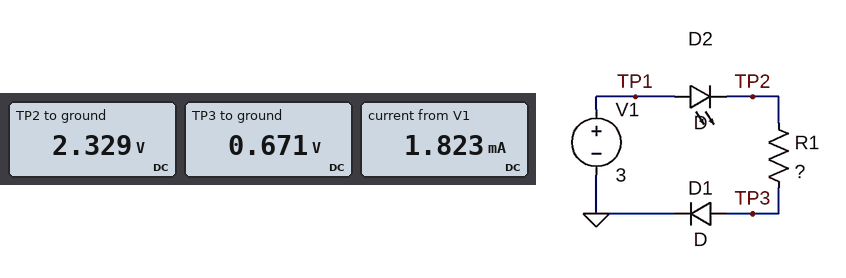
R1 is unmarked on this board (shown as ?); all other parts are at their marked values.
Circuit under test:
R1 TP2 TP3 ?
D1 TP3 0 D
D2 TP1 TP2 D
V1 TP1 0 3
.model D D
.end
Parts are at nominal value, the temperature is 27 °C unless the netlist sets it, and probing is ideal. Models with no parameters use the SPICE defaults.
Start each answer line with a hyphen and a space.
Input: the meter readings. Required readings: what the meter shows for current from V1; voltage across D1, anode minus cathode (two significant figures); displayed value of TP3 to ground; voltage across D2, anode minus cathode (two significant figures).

- 1.823 mA
- 670 mV
- 0.671 V
- 670 mV
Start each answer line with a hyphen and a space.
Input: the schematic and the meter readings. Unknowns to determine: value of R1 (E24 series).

- 910 Ω
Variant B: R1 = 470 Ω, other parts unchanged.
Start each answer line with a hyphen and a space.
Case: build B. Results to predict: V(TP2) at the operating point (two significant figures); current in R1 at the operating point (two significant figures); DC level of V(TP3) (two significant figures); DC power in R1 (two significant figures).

- 2.3 V
- 3.5 mA
- 690 mV
- 5.6 mW
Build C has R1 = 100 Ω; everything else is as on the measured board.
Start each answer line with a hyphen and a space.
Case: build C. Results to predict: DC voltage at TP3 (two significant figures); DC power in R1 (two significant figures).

- 730 mV
- 24 mW
